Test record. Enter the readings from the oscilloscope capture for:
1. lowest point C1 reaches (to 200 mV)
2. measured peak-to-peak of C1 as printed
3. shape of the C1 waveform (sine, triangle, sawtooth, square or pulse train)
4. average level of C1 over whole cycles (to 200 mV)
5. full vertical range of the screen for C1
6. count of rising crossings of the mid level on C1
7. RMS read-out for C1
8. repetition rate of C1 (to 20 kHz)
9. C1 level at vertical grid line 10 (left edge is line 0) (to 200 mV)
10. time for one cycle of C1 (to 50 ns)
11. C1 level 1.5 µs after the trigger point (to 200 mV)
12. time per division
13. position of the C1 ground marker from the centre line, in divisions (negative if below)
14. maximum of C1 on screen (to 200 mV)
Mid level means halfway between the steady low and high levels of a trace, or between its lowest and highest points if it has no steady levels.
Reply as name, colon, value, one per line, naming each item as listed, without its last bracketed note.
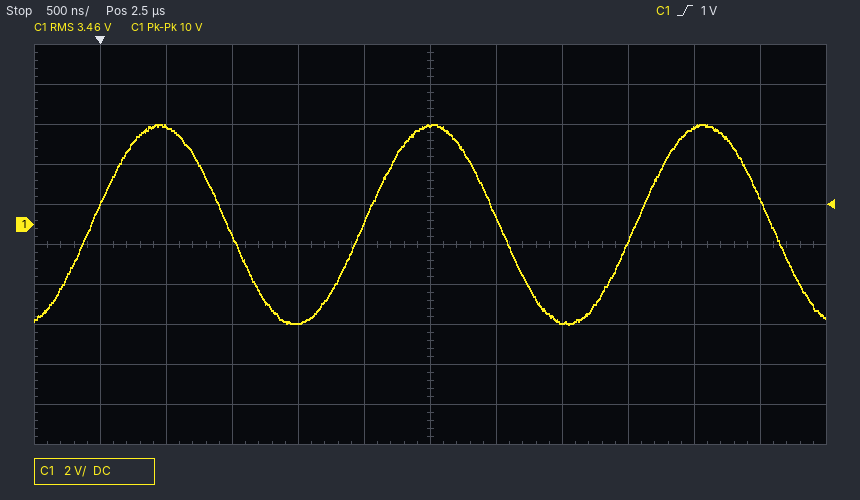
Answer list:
lowest point C1 reaches: -5.0 V
measured peak-to-peak of C1 as printed: 10 V
shape of the C1 waveform: sine
average level of C1 over whole cycles: 0.0 V
full vertical range of the screen for C1: 20 V
count of rising crossings of the mid level on C1: 3
RMS read-out for C1: 3.46 V
repetition rate of C1: 480 kHz
C1 level at vertical grid line 10 (left edge is line 0): 4.8 V
time for one cycle of C1: 2.05 µs
C1 level 1.5 µs after the trigger point: -5.0 V
time per division: 500 ns
position of the C1 ground marker from the centre line, in divisions: +0.5 div
maximum of C1 on screen: 5.0 V
